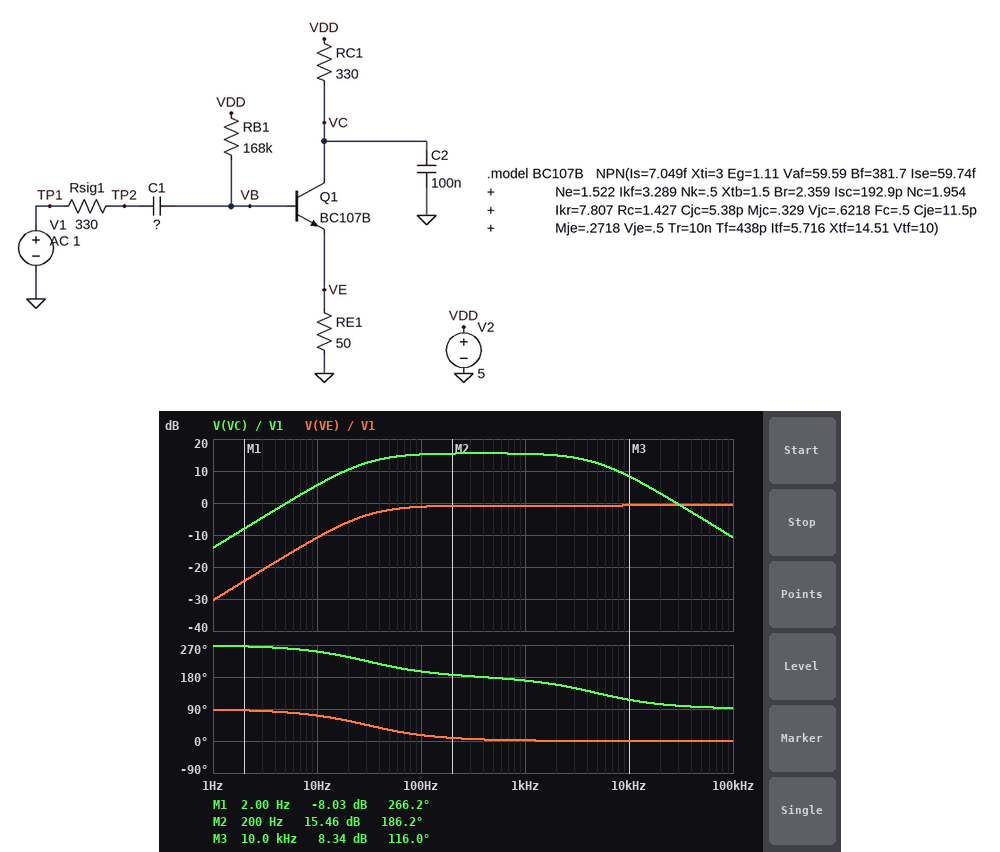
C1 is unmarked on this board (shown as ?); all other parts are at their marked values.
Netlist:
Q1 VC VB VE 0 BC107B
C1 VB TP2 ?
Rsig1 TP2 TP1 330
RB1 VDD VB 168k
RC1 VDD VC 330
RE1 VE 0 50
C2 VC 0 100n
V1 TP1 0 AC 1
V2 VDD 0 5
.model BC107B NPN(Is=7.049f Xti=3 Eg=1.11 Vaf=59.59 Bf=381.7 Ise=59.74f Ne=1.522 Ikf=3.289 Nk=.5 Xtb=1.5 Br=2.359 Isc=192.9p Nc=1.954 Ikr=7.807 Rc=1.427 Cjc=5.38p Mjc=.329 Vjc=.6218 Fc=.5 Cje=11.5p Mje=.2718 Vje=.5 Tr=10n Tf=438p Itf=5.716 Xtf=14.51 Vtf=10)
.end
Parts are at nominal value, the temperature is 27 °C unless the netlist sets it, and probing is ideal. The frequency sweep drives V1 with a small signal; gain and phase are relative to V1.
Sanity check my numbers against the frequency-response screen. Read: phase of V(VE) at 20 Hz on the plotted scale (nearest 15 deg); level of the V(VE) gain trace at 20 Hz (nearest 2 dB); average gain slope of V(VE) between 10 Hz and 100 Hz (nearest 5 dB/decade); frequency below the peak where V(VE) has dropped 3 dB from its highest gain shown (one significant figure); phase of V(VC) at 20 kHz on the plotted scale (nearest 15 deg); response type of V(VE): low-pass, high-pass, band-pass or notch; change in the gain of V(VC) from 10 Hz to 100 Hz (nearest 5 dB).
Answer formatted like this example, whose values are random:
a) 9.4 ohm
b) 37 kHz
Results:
a) 60 deg
b) -6 dB
c) 10 dB/decade
d) 30 Hz
e) 105 deg
f) high-pass
g) 10 dB
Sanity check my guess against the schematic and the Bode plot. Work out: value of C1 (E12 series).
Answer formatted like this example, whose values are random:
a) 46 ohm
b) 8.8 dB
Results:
a) 330 nF
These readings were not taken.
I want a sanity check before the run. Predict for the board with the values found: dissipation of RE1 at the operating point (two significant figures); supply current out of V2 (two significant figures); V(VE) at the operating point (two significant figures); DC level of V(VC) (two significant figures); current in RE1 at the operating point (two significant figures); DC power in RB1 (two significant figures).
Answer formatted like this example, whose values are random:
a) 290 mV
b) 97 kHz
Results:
a) 2.7 mW
b) 7.3 mA
c) 370 mV
d) 2.6 V
e) 7.3 mA
f) 91 µW
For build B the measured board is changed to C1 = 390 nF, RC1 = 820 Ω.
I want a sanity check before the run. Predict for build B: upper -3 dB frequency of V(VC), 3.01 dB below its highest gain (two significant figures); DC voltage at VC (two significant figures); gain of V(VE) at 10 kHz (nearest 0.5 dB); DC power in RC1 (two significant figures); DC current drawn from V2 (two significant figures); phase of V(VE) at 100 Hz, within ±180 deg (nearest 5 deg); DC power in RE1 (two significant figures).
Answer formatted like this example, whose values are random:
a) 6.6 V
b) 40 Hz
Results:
a) 3.8 kHz
b) 490 mV
c) -1.5 dB
d) 25 mW
e) 5.5 mA
f) 80 deg
g) 1.5 mW
